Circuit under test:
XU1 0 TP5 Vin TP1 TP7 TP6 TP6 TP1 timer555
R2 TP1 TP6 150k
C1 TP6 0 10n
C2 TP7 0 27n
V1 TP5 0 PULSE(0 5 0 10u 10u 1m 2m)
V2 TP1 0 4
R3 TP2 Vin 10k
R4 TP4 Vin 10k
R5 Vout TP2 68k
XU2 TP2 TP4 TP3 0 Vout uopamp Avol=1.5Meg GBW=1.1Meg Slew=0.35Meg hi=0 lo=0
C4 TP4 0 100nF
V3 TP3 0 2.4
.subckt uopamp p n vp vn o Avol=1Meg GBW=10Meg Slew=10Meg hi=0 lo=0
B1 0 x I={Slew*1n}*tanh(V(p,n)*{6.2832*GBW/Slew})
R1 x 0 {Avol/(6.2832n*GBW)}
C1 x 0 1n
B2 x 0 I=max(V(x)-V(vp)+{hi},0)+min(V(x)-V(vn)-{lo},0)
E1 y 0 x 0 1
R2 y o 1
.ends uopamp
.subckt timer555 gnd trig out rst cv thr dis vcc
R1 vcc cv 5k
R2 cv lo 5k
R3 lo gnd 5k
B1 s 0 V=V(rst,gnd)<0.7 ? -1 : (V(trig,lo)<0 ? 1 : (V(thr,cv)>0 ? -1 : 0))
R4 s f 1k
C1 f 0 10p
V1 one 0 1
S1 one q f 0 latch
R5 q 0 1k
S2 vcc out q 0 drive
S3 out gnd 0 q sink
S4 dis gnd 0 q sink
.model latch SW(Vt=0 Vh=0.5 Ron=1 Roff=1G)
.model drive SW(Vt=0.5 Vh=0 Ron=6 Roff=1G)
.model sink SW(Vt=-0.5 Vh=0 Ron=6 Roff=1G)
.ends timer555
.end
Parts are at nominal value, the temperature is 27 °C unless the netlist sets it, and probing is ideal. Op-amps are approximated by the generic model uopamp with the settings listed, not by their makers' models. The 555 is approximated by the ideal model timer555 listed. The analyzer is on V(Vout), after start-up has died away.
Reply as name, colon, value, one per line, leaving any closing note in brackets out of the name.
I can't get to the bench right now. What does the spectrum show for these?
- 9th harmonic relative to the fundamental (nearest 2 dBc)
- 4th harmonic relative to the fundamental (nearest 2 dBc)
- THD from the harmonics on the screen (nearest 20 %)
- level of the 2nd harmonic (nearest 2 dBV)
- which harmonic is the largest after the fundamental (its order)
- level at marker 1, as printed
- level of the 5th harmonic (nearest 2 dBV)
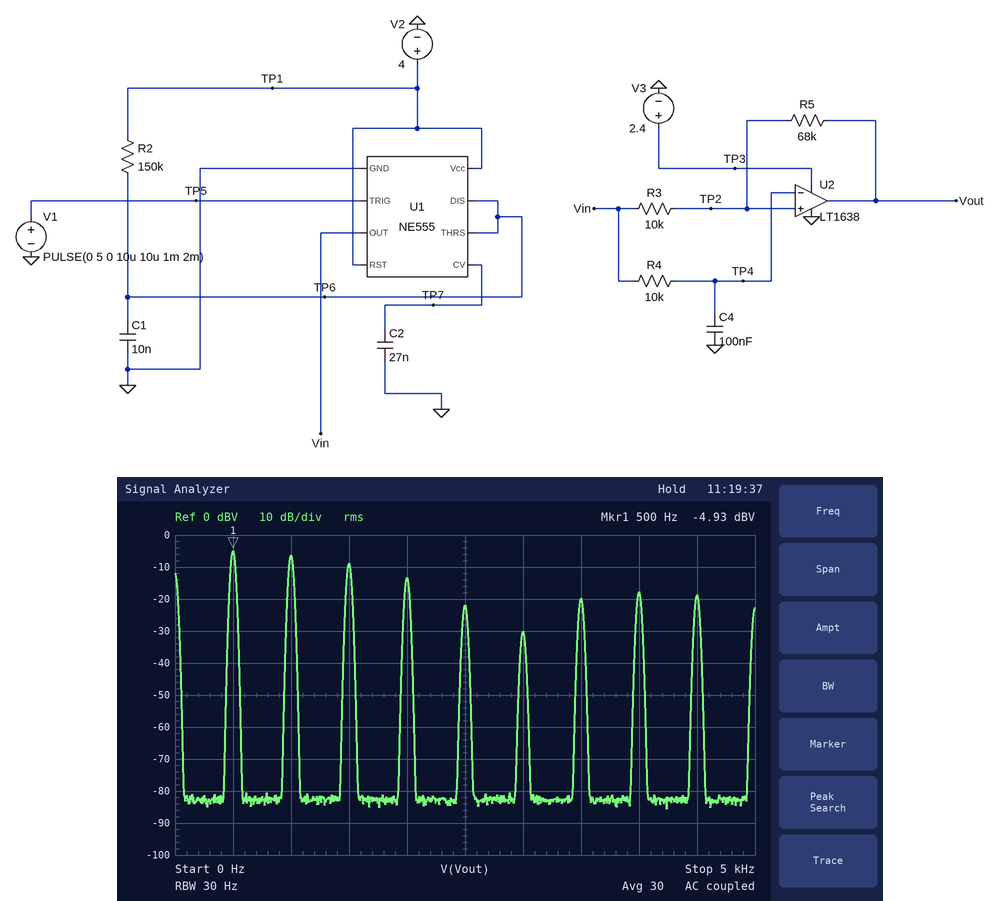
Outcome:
9th harmonic relative to the fundamental: -14 dBc
4th harmonic relative to the fundamental: -8 dBc
THD from the harmonics on the screen: 120 %
level of the 2nd harmonic: -6 dBV
which harmonic is the largest after the fundamental: 2
level at marker 1, as printed: -4.93 dBV
level of the 5th harmonic: -22 dBV
